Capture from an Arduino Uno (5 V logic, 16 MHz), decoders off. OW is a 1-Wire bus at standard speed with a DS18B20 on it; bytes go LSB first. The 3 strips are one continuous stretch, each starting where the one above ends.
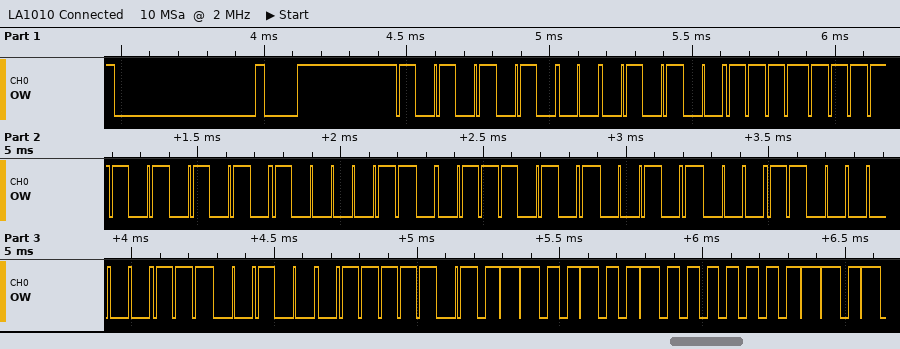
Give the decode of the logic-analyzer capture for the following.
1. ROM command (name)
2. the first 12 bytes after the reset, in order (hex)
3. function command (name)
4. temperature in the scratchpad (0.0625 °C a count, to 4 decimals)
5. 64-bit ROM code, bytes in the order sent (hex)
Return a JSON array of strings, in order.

["Match ROM", "55 28 FF 55 61 AE 14 03 27 BE 26 01", "Read Scratchpad", "18.3750 °C", "28 FF 55 61 AE 14 03 27"]
